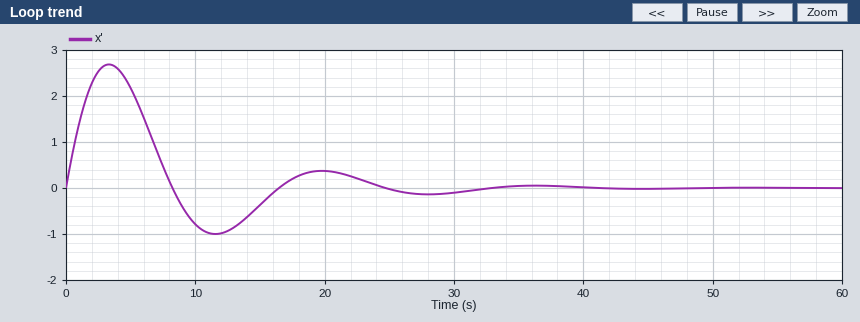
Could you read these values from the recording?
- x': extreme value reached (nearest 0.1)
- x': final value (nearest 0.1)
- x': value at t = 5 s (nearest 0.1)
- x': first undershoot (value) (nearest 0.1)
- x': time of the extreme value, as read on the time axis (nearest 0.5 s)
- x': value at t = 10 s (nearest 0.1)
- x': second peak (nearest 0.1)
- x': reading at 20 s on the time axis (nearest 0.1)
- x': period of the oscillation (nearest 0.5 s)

2.7
0.0
2.2
-1.0
3.5 s
-0.8
0.4
0.4
16.5 s
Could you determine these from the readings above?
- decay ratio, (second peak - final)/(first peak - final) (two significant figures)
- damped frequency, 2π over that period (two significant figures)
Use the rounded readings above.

0.15
0.38 rad/s
